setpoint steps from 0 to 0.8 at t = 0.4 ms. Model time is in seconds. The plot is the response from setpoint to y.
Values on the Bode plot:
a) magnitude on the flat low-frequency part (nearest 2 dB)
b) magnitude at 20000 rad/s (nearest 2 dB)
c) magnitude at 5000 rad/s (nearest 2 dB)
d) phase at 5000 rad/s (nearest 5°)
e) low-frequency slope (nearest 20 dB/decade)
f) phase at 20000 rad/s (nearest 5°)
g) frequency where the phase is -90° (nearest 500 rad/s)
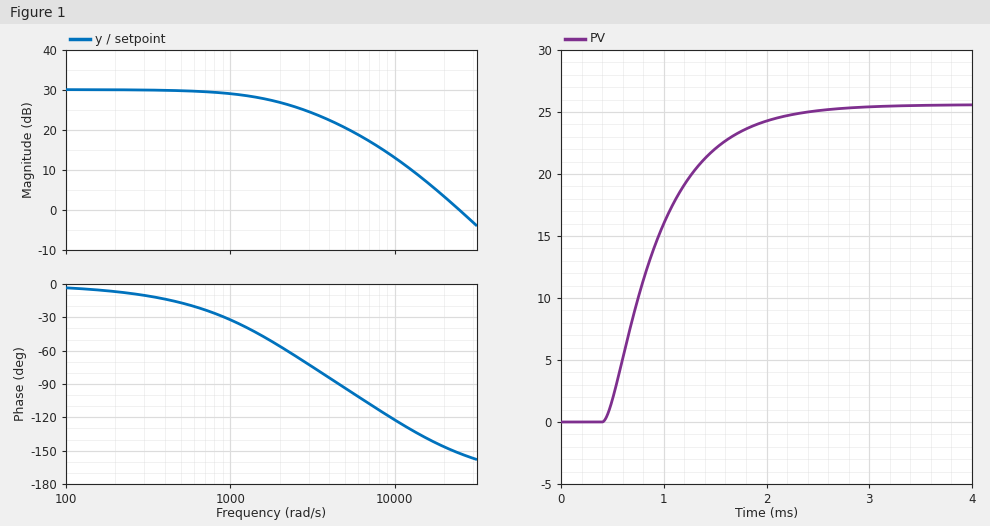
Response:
30 dB
4 dB
20 dB
-95°
0 dB/decade
-145°
4500 rad/s
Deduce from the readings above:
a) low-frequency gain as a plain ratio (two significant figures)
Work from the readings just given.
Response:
32
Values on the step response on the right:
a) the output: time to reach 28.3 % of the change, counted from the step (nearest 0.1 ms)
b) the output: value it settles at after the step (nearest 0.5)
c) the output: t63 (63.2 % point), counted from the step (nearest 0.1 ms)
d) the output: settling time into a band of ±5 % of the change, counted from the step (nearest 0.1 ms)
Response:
0.3 ms
25.5
0.6 ms
1.6 ms
